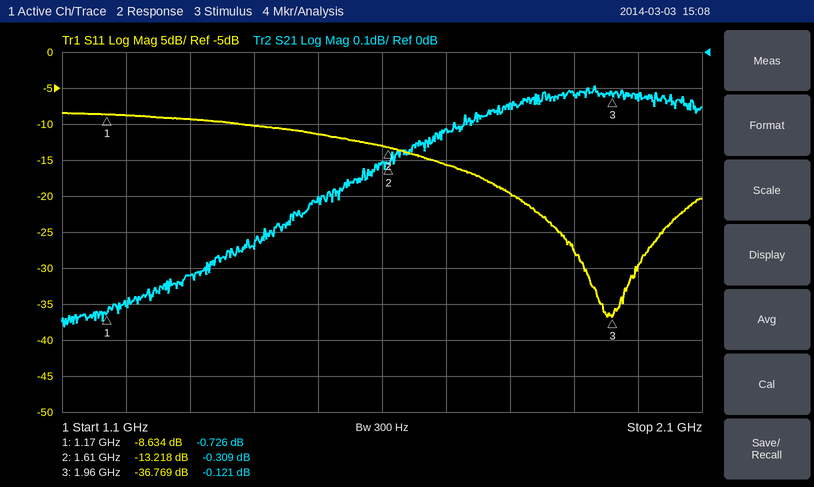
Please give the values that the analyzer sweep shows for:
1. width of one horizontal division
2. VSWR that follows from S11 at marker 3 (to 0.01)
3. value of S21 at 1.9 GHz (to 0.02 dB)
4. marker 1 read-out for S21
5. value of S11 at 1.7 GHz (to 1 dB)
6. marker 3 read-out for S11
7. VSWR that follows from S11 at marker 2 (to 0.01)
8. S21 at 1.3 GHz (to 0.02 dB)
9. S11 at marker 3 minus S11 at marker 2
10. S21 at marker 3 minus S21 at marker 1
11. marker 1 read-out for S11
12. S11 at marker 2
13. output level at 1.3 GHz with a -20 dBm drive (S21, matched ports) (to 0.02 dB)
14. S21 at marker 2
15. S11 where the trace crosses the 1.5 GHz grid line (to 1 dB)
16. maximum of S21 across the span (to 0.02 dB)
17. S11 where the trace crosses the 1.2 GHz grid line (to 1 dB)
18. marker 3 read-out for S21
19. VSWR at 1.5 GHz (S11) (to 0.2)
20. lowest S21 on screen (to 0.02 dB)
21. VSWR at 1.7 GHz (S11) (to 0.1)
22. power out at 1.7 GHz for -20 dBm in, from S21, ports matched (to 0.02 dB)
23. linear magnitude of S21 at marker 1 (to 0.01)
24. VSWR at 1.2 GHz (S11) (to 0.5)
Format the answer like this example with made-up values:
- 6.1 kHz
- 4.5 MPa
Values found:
- 100 MHz
- 1.03
- -0.12 dB
- -0.726 dB
- -16 dB
- -36.769 dB
- 1.56
- -0.62 dB
- -23.551 dB
- 0.605 dB
- -8.634 dB
- -13.218 dB
- -20.62 dBm
- -0.309 dB
- -11 dB
- -0.10 dB
- -9 dB
- -0.121 dB
- 1.8
- -0.76 dB
- 1.4
- -20.22 dBm
- 0.92
- 2.0
